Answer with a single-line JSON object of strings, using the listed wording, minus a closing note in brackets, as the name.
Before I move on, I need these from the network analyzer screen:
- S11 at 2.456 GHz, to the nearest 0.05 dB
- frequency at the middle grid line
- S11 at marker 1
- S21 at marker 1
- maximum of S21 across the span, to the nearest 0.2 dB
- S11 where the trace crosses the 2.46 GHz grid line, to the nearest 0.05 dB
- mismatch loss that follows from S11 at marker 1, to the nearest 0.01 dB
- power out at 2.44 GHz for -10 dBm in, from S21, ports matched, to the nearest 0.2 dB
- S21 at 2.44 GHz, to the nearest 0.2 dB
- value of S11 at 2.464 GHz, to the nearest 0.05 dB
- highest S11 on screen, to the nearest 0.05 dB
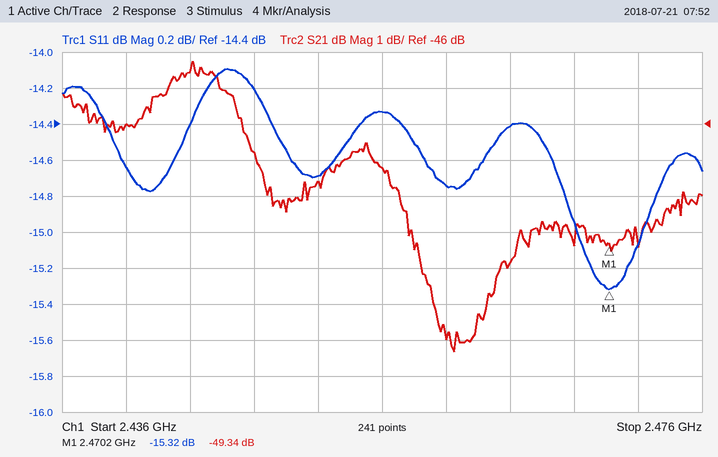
{"S11 at 2.456 GHz, to the nearest 0.05 dB": "-14.35 dB", "frequency at the middle grid line": "2.456 GHz", "S11 at marker 1": "-15.32 dB", "S21 at marker 1": "-49.34 dB", "maximum of S21 across the span, to the nearest 0.2 dB": "-44.2 dB", "S11 where the trace crosses the 2.46 GHz grid line, to the nearest 0.05 dB": "-14.75 dB", "mismatch loss that follows from S11 at marker 1, to the nearest 0.01 dB": "0.13 dB", "power out at 2.44 GHz for -10 dBm in, from S21, ports matched, to the nearest 0.2 dB": "-56.0 dBm", "S21 at 2.44 GHz, to the nearest 0.2 dB": "-46.0 dB", "value of S11 at 2.464 GHz, to the nearest 0.05 dB": "-14.40 dB", "highest S11 on screen, to the nearest 0.05 dB": "-14.10 dB"}
